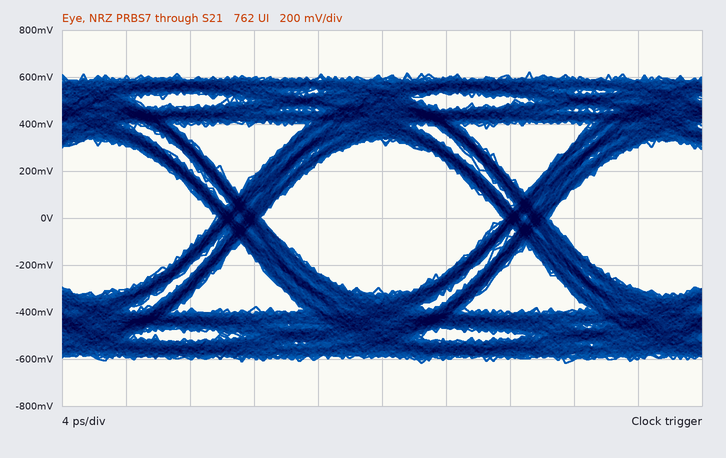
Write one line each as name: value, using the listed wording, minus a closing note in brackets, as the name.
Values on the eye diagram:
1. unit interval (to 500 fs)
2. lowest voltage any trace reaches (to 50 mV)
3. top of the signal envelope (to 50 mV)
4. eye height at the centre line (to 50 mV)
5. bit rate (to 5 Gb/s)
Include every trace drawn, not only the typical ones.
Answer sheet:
unit interval: 18.0 ps
lowest voltage any trace reaches: -600 mV
top of the signal envelope: 600 mV
eye height at the centre line: 650 mV
bit rate: 55 Gb/s
